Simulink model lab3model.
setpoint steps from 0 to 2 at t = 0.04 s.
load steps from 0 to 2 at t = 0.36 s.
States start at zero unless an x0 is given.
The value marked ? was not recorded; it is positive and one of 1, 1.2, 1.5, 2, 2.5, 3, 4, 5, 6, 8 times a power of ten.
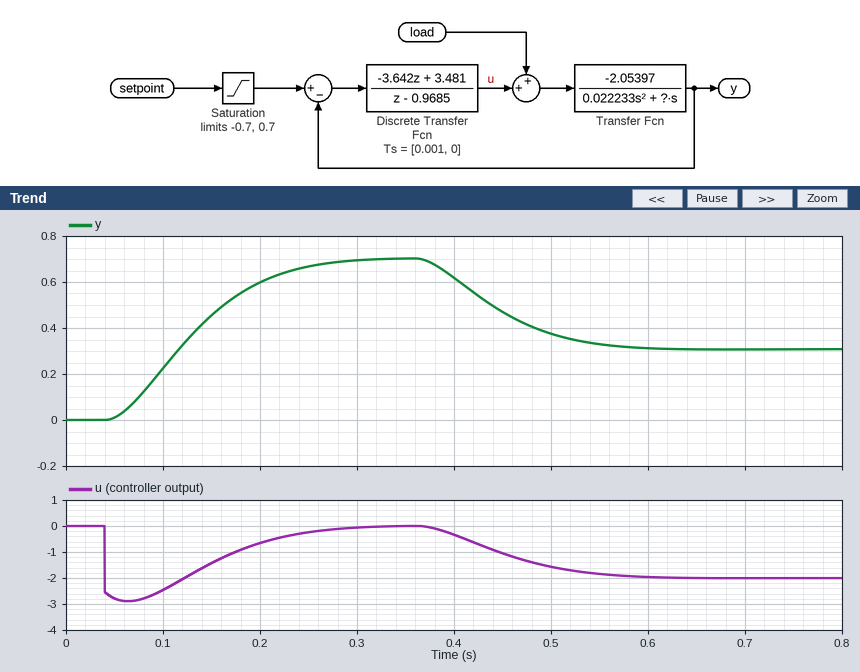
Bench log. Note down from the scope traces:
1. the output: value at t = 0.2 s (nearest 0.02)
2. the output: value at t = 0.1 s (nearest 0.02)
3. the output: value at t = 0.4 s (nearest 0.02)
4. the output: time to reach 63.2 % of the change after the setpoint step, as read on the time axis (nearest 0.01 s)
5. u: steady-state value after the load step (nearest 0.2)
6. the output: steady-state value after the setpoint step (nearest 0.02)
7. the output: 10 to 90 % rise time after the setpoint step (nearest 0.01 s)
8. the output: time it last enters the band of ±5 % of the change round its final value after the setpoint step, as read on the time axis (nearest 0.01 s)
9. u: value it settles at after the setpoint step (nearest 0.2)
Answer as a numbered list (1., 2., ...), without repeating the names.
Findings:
1. 0.60
2. 0.22
3. 0.62
4. 0.15 s
5. -2.0
6. 0.70
7. 0.15 s
8. 0.25 s
9. 0.0
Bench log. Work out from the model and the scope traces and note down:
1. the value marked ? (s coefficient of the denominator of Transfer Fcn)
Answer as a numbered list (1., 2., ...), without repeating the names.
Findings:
1. 1
